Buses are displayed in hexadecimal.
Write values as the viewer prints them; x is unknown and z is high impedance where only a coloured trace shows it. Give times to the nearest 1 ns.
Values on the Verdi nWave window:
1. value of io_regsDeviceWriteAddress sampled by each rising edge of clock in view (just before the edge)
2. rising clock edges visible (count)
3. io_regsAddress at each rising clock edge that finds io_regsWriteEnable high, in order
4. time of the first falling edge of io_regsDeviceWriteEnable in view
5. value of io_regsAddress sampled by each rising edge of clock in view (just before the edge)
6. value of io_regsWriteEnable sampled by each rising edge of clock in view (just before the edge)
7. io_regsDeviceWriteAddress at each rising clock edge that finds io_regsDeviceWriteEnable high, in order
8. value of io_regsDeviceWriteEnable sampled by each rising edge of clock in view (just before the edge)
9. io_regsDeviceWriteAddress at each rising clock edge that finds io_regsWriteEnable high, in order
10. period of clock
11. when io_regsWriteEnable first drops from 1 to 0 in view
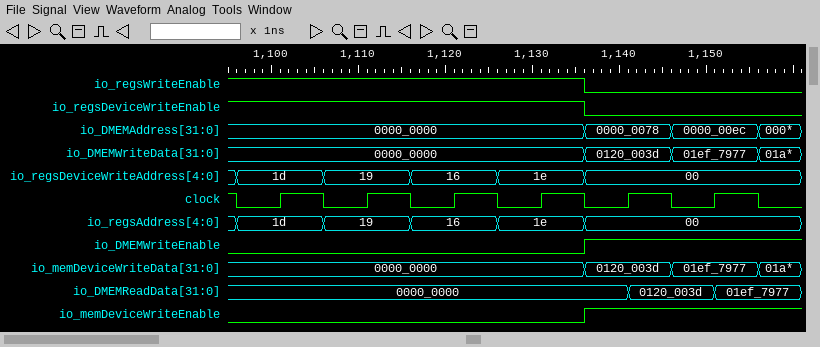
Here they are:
1d, 19, 16, 1e, 00, 00
6
1d, 19, 16, 1e
1136 ns
1d, 19, 16, 1e, 00, 00
1 1 1 1 0 0
1d, 19, 16, 1e
1 1 1 1 0 0
1d, 19, 16, 1e
10 ns
1136 ns
